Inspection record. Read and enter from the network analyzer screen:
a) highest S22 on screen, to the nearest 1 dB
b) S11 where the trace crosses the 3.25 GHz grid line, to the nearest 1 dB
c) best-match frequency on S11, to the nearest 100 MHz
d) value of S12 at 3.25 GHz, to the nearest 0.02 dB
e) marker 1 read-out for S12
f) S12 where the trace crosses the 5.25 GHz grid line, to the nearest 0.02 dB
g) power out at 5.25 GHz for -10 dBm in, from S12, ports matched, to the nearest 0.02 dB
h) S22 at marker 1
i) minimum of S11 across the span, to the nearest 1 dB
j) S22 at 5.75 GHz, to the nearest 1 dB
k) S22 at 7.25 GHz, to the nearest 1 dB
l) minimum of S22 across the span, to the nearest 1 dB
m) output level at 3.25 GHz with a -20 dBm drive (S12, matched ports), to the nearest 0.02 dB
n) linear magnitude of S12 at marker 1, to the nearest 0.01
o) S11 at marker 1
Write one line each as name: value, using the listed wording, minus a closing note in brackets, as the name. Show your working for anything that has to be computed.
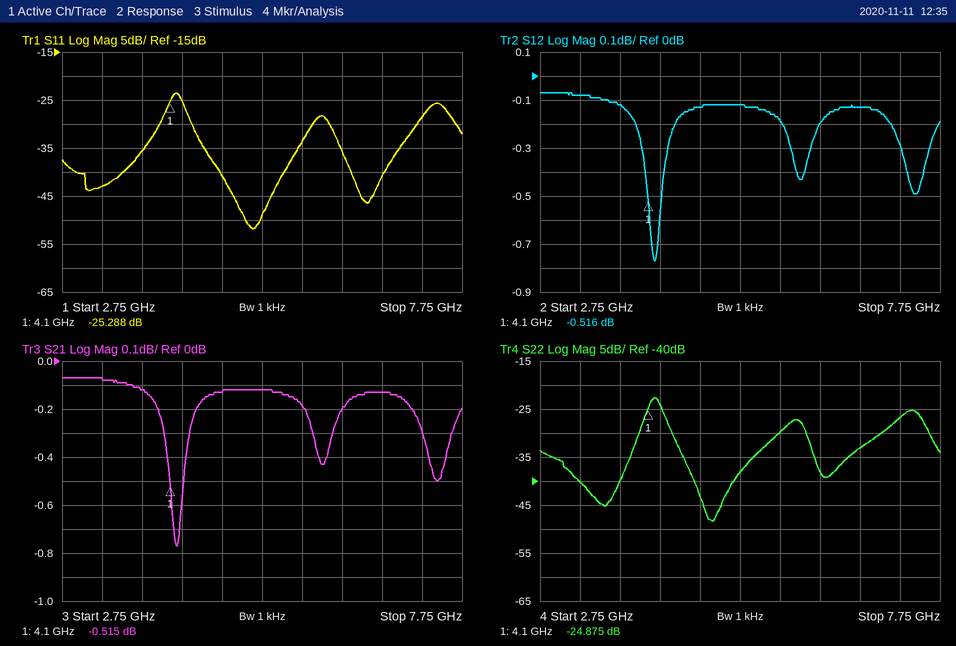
highest S22 on screen, to the nearest 1 dB: -23 dB
S11 where the trace crosses the 3.25 GHz grid line, to the nearest 1 dB: -43 dB
best-match frequency on S11, to the nearest 100 MHz: 5.1 GHz
value of S12 at 3.25 GHz, to the nearest 0.02 dB: -0.08 dB
marker 1 read-out for S12: -0.516 dB
S12 where the trace crosses the 5.25 GHz grid line, to the nearest 0.02 dB: -0.12 dB
power out at 5.25 GHz for -10 dBm in, from S12, ports matched, to the nearest 0.02 dB: -10 dBm + (-0.12 dB) = -10.12 dBm
S22 at marker 1: -24.875 dB
minimum of S11 across the span, to the nearest 1 dB: -52 dB
S22 at 5.75 GHz, to the nearest 1 dB: -30 dB
S22 at 7.25 GHz, to the nearest 1 dB: -27 dB
minimum of S22 across the span, to the nearest 1 dB: -48 dB
output level at 3.25 GHz with a -20 dBm drive (S12, matched ports), to the nearest 0.02 dB: -20 dBm + (-0.08 dB) = -20.08 dBm
linear magnitude of S12 at marker 1, to the nearest 0.01: 10^(-0.516/20) ≈ 0.94
S11 at marker 1: -25.288 dB
